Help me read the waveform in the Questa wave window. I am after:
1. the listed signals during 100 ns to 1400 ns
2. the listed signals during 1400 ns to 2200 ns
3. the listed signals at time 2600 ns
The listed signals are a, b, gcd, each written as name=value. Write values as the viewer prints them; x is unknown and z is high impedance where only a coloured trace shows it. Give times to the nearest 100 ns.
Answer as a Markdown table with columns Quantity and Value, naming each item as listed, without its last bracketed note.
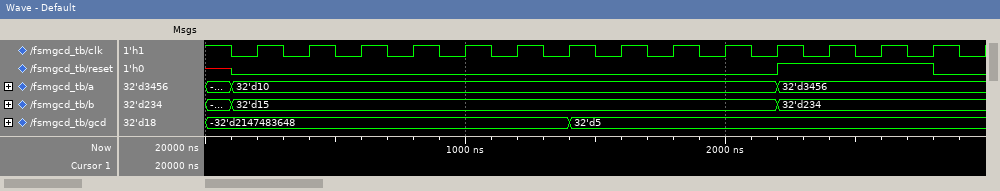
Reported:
| Quantity | Value |
|---|---|
| the listed signals during 100 ns to 1400 ns | a=32'd10, b=32'd15, gcd=-32'd2147483648 |
| the listed signals during 1400 ns to 2200 ns | a=32'd10, b=32'd15, gcd=32'd5 |
| the listed signals at time 2600 ns | a=32'd3456, b=32'd234, gcd=32'd5 |
